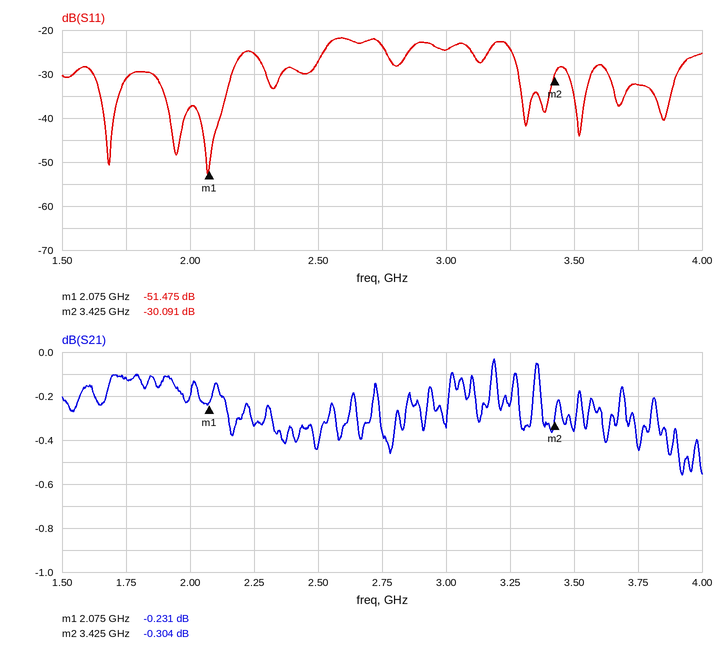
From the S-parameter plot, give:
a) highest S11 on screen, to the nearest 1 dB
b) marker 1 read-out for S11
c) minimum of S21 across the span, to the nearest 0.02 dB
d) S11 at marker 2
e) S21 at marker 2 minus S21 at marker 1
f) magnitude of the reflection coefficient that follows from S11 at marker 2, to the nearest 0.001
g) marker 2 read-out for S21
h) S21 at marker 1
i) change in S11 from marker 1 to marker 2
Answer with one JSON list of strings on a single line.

["-22 dB", "-51.475 dB", "-0.56 dB", "-30.091 dB", "-0.073 dB", "0.031", "-0.304 dB", "-0.231 dB", "21.384 dB"]
